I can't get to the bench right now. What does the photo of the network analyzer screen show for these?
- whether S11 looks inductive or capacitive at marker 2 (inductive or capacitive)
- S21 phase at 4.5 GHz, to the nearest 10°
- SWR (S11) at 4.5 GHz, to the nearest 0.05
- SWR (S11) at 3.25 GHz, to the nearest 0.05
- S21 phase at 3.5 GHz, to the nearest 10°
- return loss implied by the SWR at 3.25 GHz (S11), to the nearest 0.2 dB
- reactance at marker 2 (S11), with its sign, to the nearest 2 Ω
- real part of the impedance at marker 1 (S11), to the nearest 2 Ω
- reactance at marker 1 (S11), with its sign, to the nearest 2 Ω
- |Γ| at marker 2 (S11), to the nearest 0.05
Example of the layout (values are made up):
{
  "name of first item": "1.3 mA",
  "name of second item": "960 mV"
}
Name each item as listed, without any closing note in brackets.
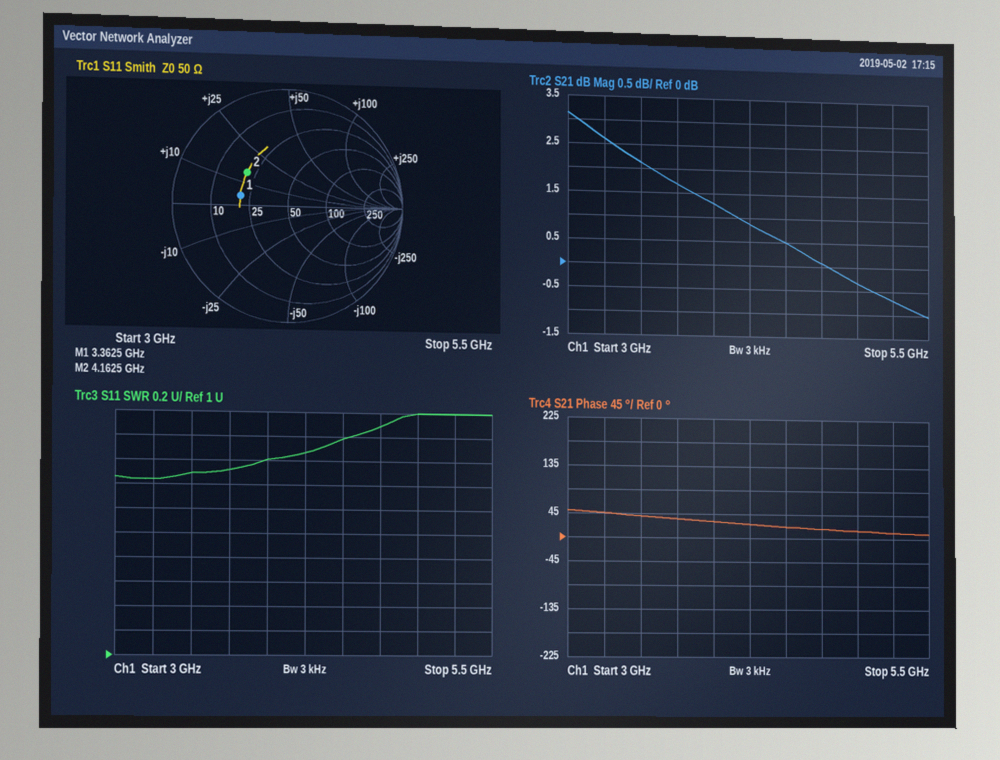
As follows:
{
  "whether S11 looks inductive or capacitive at marker 2": "inductive",
  "S21 phase at 4.5 GHz, to the nearest 10°": "20°",
  "SWR (S11) at 4.5 GHz, to the nearest 0.05": "2.80",
  "SWR (S11) at 3.25 GHz, to the nearest 0.05": "2.45",
  "S21 phase at 3.5 GHz, to the nearest 10°": "40°",
  "return loss implied by the SWR at 3.25 GHz (S11), to the nearest 0.2 dB": "7.6 dB",
  "reactance at marker 2 (S11), with its sign, to the nearest 2 Ω": "+14 Ω",
  "real part of the impedance at marker 1 (S11), to the nearest 2 Ω": "20 Ω",
  "reactance at marker 1 (S11), with its sign, to the nearest 2 Ω": "+4 Ω",
  "|Γ| at marker 2 (S11), to the nearest 0.05": "0.45"
}
